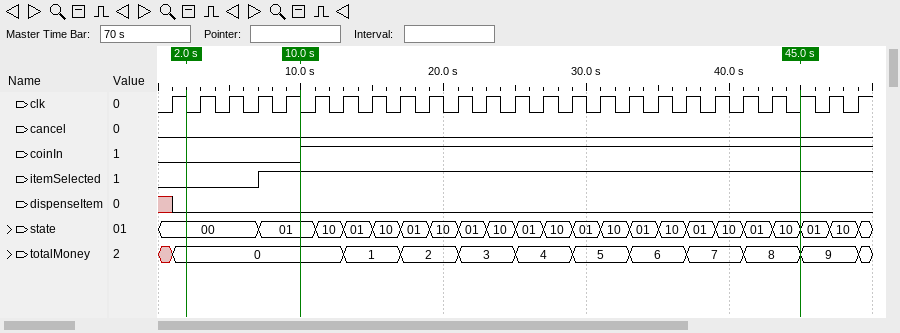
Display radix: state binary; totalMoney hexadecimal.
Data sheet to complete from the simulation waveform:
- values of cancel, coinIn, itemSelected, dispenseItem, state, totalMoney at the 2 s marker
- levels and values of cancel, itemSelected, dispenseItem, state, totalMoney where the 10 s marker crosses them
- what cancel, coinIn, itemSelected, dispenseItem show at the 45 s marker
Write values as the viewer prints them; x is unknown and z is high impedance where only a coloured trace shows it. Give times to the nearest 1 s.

cancel=0, coinIn=0, itemSelected=0, dispenseItem=0, state=00, totalMoney=0
cancel=0, itemSelected=1, dispenseItem=0, state=01, totalMoney=0
cancel=0, coinIn=1, itemSelected=1, dispenseItem=0
